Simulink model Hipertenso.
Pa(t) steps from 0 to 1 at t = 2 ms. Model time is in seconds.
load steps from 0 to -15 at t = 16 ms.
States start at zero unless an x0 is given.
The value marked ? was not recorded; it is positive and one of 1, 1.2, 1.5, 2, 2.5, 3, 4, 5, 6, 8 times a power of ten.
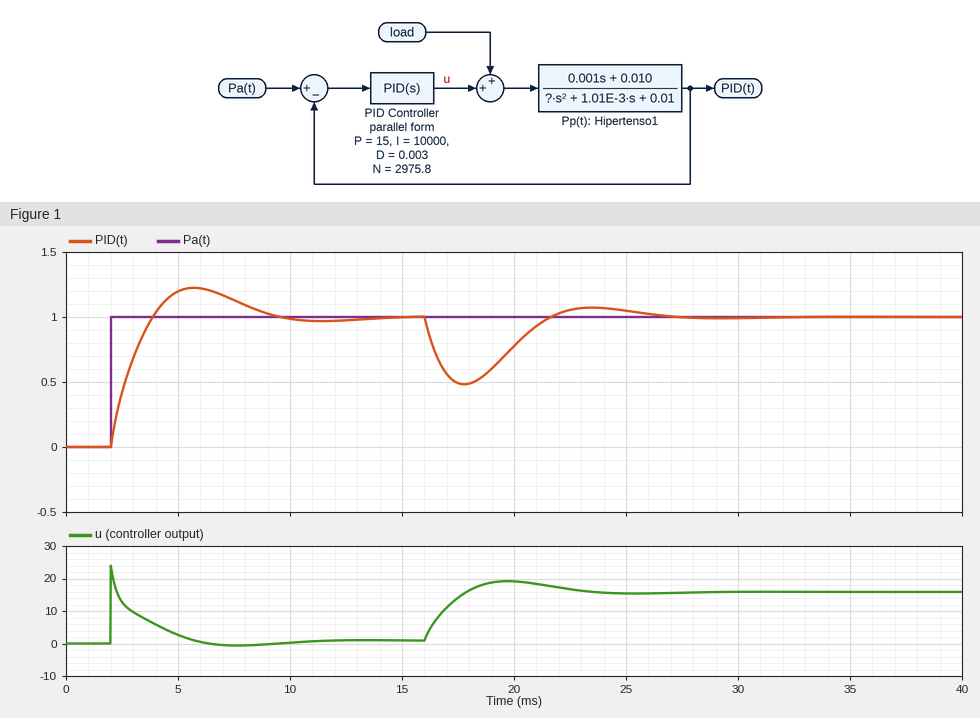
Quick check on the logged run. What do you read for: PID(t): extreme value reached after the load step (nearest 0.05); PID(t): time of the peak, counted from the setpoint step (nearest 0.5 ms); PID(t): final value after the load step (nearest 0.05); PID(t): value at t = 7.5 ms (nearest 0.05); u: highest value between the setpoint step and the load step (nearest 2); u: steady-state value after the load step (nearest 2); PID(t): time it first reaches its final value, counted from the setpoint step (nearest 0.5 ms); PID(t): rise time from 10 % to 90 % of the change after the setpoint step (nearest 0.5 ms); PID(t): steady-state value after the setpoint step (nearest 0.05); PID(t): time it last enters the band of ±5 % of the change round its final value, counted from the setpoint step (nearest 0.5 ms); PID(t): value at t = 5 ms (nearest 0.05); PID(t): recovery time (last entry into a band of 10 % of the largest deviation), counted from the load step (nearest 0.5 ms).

0.50
3.5 ms
1.00
1.15
24
16
2.0 ms
1.5 ms
1.00
6.5 ms
1.20
9.0 ms
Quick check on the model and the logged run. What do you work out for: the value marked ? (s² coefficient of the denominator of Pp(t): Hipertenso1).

2e-05
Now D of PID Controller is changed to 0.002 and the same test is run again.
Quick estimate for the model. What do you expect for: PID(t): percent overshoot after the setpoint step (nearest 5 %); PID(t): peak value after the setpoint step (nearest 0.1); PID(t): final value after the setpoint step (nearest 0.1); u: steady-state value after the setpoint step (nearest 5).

25 %
1.2
1.0
0
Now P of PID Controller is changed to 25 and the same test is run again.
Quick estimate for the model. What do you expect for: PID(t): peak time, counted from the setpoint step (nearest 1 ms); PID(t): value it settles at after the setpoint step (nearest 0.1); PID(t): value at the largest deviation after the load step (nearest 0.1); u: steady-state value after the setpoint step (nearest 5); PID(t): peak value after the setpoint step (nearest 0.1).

3 ms
1.0
0.6
0
1.1
